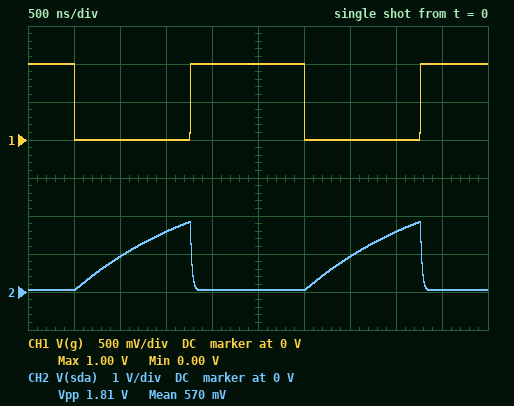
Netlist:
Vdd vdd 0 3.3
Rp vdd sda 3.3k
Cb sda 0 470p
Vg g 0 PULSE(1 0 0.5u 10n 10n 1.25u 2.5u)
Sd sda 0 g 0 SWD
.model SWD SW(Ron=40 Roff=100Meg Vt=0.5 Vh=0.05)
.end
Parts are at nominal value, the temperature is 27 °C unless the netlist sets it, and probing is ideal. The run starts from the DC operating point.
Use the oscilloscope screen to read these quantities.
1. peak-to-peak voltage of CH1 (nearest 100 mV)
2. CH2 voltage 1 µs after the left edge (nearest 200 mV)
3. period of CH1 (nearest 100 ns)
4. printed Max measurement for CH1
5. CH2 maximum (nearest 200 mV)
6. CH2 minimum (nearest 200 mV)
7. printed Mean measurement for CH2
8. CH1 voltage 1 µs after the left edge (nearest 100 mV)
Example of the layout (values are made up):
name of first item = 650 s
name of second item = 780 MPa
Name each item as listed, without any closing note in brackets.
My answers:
peak-to-peak voltage of CH1 = 1.0 V
CH2 voltage 1 µs after the left edge = 1.0 V
period of CH1 = 2.5 µs
printed Max measurement for CH1 = 1.00 V
CH2 maximum = 1.8 V
CH2 minimum = 0 V
printed Mean measurement for CH2 = 570 mV
CH1 voltage 1 µs after the left edge = 0 V
